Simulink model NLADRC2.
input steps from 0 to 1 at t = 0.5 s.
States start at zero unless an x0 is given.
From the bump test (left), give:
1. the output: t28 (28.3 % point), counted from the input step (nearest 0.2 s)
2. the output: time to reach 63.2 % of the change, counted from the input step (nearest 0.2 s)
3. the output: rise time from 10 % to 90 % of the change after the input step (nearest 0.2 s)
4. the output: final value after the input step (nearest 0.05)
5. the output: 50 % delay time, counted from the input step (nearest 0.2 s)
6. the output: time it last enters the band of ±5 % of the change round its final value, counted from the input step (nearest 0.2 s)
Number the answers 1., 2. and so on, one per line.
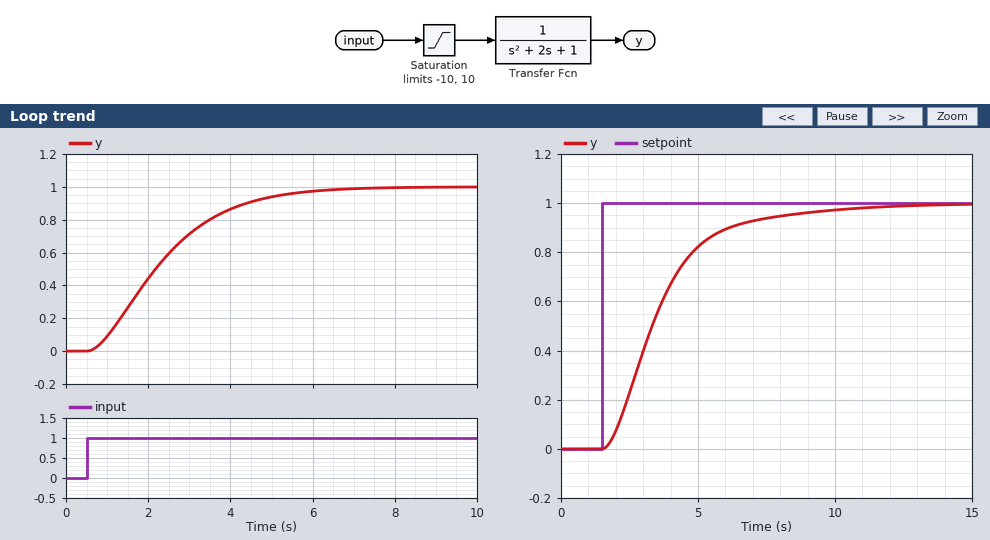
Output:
1. 1.0 s
2. 2.2 s
3. 3.4 s
4. 1.00
5. 1.6 s
6. 4.8 s
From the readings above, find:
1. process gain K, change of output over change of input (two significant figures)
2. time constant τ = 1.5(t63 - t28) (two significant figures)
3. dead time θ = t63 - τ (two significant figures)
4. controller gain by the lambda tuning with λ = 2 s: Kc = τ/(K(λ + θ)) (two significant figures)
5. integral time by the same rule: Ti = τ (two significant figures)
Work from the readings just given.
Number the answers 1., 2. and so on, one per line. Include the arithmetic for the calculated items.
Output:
1. (1 - 0) / 1 = 1.0
2. 1.5 × (2.2 - 1) = 1.8 s
3. 2.2 - 1.8 = 0.40 s
4. 1.8 / (1 × (2 + 0.4)) = 0.75
5. 1.8 s
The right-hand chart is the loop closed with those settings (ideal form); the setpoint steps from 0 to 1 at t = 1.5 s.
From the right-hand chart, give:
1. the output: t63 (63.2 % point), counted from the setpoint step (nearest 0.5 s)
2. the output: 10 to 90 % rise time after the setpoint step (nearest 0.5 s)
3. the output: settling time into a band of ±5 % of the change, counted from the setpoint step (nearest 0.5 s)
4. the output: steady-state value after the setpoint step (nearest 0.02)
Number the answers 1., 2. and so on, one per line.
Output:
1. 2.5 s
2. 4.0 s
3. 6.5 s
4. 1.00
